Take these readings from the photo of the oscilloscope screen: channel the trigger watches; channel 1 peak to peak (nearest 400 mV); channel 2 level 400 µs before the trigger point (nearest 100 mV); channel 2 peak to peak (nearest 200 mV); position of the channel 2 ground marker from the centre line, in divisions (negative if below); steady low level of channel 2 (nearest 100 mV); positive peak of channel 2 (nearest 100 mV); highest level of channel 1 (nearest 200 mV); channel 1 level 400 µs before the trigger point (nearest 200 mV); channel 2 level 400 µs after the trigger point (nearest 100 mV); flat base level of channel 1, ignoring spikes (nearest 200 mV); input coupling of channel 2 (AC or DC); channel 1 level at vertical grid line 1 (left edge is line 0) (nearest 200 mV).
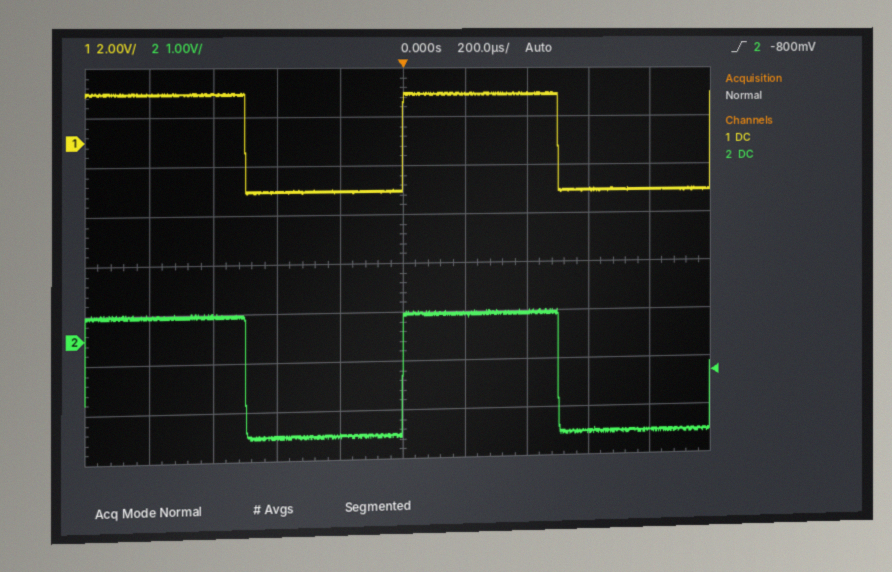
channel 2
4.0 V
-2.0 V
2.6 V
-1.5 div
-2.0 V
500 mV
2.0 V
-2.0 V
500 mV
-2.0 V
DC
2.0 V
